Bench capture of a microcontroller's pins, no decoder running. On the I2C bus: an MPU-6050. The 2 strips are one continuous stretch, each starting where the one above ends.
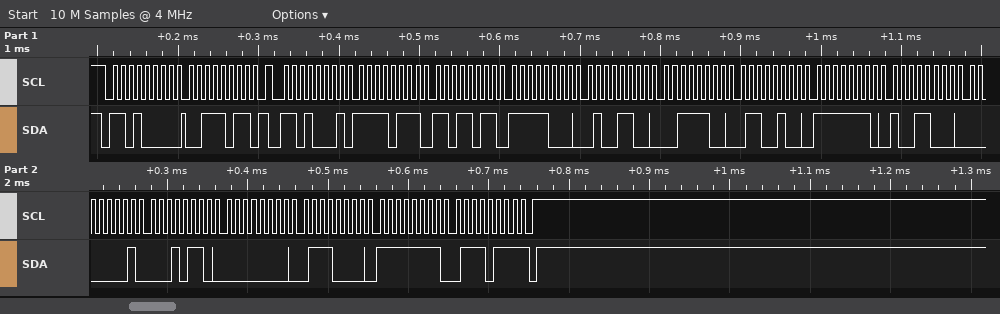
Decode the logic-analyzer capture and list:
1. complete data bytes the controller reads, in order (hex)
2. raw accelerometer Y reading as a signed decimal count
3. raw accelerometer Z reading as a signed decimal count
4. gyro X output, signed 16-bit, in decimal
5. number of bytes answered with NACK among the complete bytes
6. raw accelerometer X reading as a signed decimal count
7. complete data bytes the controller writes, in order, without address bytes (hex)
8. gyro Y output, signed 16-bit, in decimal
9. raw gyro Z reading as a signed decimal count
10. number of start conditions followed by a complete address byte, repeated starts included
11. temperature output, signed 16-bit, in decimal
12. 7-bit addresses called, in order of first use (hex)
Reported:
F7 DB F8 4C 3C 64 FE 98 01 16 00 70 FF 77
-1972
15460
278
1
-2085
3B
112
-137
2
-360
0x68
